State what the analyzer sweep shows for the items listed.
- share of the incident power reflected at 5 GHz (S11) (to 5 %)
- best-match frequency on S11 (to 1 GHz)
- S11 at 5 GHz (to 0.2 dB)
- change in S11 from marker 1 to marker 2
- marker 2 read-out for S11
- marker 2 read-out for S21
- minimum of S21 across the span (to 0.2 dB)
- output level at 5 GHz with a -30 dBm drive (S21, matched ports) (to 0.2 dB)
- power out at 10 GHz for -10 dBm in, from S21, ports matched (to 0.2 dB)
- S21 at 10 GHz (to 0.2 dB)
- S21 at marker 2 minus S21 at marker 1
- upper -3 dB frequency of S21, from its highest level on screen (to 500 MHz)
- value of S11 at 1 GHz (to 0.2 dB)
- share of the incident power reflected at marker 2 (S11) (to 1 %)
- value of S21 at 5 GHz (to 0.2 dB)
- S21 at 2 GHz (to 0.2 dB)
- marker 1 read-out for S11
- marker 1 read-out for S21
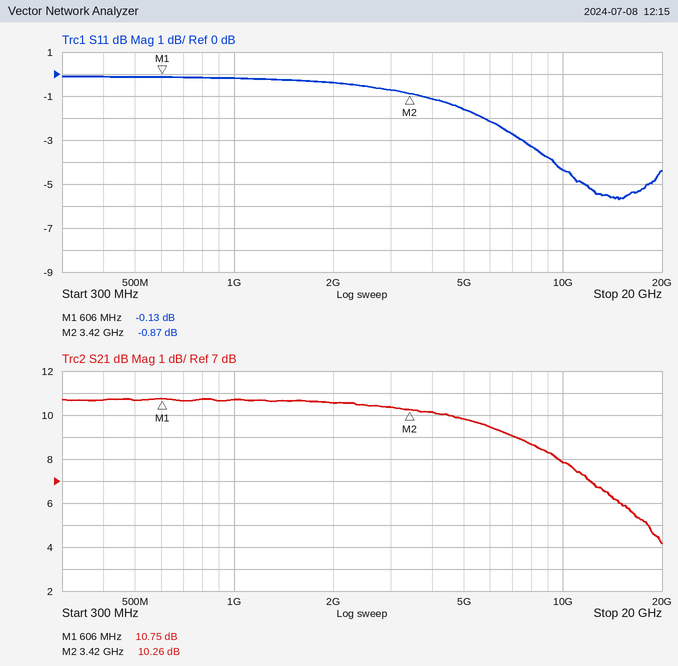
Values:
70 %
15 GHz
-1.6 dB
-0.74 dB
-0.87 dB
10.26 dB
4.2 dB
-20.2 dBm
-2.2 dBm
7.8 dB
-0.49 dB
10.5 GHz
-0.2 dB
82 %
9.8 dB
10.6 dB
-0.13 dB
10.75 dB
